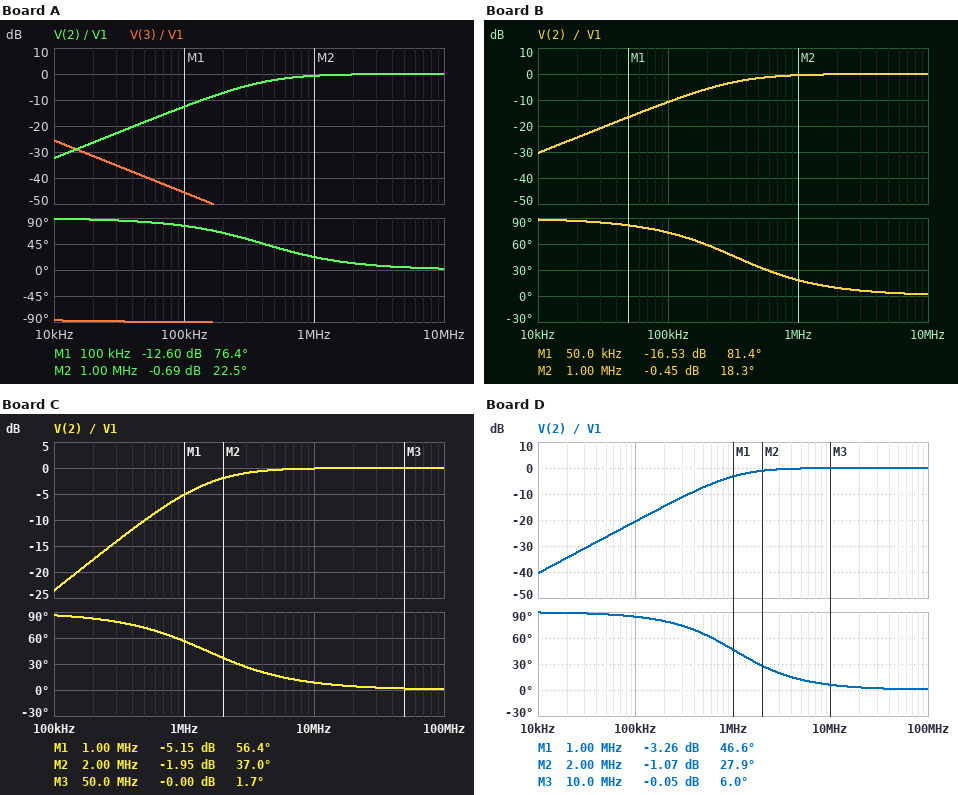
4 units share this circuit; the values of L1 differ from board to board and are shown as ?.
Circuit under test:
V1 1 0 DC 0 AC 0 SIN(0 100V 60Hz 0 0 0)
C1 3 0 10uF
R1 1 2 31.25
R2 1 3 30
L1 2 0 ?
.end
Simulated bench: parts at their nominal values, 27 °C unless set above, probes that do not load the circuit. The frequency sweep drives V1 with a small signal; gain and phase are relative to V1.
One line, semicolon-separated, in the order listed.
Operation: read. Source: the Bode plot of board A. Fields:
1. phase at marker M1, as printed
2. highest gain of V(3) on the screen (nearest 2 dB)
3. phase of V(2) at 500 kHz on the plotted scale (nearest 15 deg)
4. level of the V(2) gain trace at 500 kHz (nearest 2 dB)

76.4 deg; -26 dB; 45 deg; -2 dB
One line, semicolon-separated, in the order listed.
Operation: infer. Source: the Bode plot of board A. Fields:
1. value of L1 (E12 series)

12 µH
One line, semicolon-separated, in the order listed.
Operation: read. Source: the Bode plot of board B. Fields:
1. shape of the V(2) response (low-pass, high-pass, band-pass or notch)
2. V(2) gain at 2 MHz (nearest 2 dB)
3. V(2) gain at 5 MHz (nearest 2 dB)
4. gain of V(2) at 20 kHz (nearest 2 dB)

high-pass; 0 dB; 0 dB; -24 dB
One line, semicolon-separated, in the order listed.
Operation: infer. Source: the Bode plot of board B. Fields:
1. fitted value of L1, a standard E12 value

15 µH
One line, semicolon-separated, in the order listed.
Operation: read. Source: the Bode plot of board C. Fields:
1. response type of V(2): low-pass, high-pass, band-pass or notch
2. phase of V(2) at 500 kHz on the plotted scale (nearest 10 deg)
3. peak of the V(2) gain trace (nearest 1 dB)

high-pass; 70 deg; 0 dB
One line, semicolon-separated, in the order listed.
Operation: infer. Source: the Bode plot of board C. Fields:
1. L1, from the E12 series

3.3 µH
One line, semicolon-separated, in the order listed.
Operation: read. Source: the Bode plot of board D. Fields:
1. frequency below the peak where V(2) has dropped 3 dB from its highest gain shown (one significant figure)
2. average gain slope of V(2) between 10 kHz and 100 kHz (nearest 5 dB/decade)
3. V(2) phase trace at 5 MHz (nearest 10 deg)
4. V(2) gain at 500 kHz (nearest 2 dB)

1 MHz; 20 dB/decade; 10 deg; -8 dB
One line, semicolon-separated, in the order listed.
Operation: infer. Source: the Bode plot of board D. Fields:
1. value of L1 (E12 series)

4.7 µH
